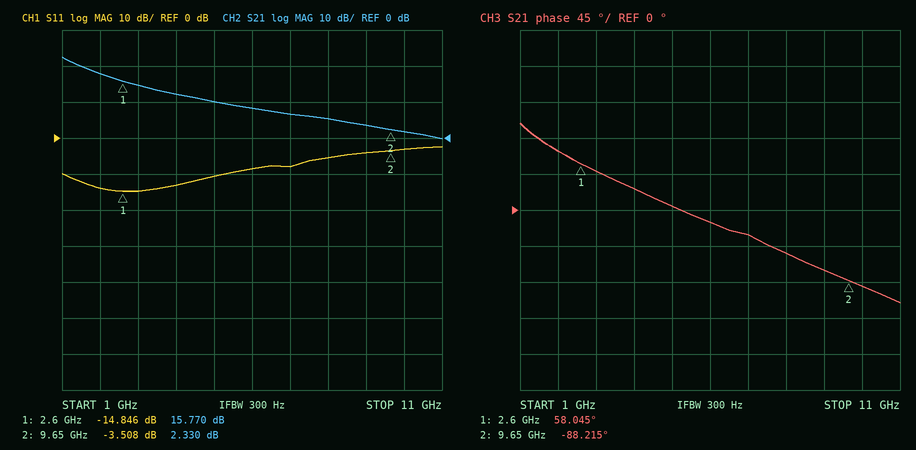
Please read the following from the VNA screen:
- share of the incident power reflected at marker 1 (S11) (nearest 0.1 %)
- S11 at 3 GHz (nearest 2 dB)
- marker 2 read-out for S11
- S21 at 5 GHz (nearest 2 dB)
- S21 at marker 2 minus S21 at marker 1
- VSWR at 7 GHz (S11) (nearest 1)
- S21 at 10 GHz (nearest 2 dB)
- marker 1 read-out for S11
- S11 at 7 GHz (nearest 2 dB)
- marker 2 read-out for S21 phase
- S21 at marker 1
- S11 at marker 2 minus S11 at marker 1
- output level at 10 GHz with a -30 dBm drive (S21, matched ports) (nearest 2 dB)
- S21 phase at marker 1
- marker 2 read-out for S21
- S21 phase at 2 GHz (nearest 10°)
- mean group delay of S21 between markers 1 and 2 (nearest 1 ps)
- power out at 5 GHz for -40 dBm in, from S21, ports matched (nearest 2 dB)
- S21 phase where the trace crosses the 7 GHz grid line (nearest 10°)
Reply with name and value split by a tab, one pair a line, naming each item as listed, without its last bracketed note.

share of the incident power reflected at marker 1 (S11)	3.3 %
S11 at 3 GHz	-14 dB
marker 2 read-out for S11	-3.508 dB
S21 at 5 GHz	10 dB
S21 at marker 2 minus S21 at marker 1	-13.440 dB
VSWR at 7 GHz (S11)	2
S21 at 10 GHz	2 dB
marker 1 read-out for S11	-14.846 dB
S11 at 7 GHz	-8 dB
marker 2 read-out for S21 phase	-88.215°
S21 at marker 1	15.770 dB
S11 at marker 2 minus S11 at marker 1	11.338 dB
output level at 10 GHz with a -30 dBm drive (S21, matched ports)	-28 dBm
S21 phase at marker 1	58.045°
marker 2 read-out for S21	2.330 dB
S21 phase at 2 GHz	70°
mean group delay of S21 between markers 1 and 2	58 ps
power out at 5 GHz for -40 dBm in, from S21, ports matched	-30 dBm
S21 phase where the trace crosses the 7 GHz grid line	-30°
